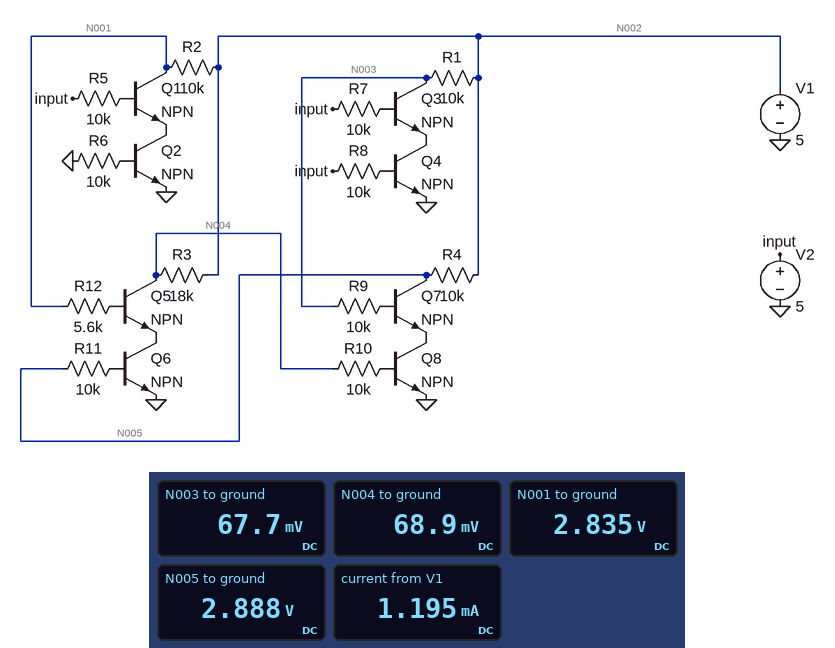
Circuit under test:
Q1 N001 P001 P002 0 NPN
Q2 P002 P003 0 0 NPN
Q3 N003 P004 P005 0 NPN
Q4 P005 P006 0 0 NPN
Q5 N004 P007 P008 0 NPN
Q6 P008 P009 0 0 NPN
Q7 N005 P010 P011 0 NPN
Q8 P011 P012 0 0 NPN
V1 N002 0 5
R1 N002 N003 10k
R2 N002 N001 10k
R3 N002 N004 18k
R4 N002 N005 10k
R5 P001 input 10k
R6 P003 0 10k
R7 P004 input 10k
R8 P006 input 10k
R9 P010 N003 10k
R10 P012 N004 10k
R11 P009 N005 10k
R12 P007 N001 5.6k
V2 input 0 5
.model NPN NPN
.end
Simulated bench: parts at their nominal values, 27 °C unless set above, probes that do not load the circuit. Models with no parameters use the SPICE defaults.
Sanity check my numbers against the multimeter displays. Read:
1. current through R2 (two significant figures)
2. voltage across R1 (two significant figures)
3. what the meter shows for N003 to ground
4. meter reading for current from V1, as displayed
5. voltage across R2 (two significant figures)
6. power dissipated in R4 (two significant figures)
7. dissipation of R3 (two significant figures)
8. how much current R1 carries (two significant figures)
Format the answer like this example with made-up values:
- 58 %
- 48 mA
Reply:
- 220 µA
- 4.9 V
- 67.7 mV
- 1.195 mA
- 2.2 V
- 450 µW
- 1.4 mW
- 490 µA
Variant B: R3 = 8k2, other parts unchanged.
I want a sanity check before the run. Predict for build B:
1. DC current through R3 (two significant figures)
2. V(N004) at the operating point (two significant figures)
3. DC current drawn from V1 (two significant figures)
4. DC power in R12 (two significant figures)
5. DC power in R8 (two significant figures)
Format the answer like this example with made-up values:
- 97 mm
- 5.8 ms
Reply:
- 600 µA
- 84 mV
- 1.5 mA
- 720 µW
- 1.8 mW
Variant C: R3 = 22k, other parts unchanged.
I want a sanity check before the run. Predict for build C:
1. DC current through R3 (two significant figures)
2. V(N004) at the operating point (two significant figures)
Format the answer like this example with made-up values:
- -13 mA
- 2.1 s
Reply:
- 220 µA
- 66 mV
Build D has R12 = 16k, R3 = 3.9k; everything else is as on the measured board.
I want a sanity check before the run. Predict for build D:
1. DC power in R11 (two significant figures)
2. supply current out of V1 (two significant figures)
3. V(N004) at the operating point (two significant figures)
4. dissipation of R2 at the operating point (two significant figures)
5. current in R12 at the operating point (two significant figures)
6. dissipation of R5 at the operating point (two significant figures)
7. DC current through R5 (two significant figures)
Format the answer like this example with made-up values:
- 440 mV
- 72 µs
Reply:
- 440 µW
- 2.1 mA
- 120 mV
- 160 µW
- 180 µA
- 31 µW
- 56 µA
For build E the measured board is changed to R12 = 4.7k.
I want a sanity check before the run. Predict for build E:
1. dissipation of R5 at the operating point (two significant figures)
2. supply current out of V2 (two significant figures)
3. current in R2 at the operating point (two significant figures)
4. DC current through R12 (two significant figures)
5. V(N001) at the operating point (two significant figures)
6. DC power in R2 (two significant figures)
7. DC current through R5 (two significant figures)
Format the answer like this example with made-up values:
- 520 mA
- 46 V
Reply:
- 260 µW
- 1.0 mA
- 230 µA
- 390 µA
- 2.7 V
- 540 µW
- 160 µA
